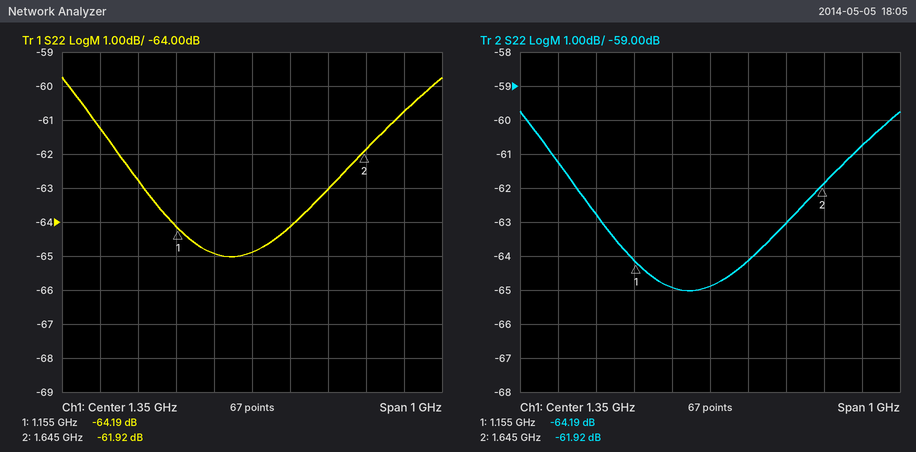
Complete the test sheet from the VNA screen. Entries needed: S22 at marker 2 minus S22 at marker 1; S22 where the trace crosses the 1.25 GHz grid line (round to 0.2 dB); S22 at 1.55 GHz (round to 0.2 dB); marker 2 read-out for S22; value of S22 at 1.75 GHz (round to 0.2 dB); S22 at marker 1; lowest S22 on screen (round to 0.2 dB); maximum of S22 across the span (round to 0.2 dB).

2.27 dB
-65.0 dB
-63.0 dB
-61.92 dB
-60.8 dB
-64.19 dB
-65.0 dB
-59.8 dB
